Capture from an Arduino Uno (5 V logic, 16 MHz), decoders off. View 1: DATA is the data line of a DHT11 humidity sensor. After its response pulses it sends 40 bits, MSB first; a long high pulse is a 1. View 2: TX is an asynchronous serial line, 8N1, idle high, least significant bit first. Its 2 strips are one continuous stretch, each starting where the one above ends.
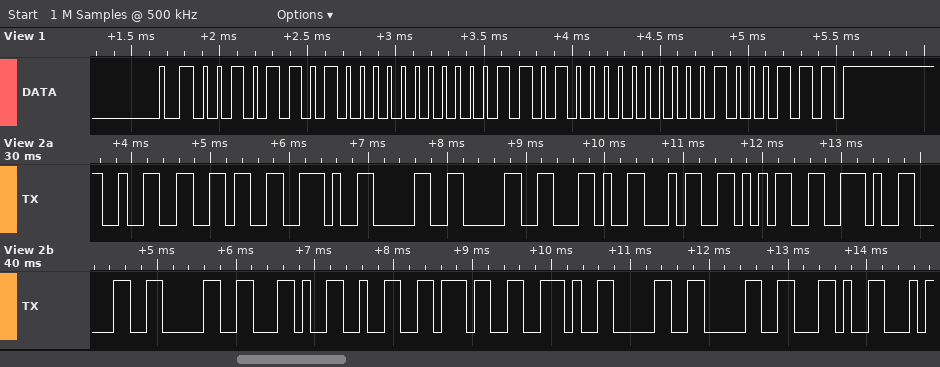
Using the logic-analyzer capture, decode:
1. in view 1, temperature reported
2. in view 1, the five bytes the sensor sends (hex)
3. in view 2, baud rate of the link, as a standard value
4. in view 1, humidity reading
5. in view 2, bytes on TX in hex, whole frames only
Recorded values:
26.0 °C
2D 00 1A 00 47
9600 baud
45 %
0x32 0x36 0x2E 0x30 0x30 0x2C 0x34 0x35 0x2E 0x30 0x30 0x2C 0x32 0x37 0x2E 0x30 0x30 0x2C
